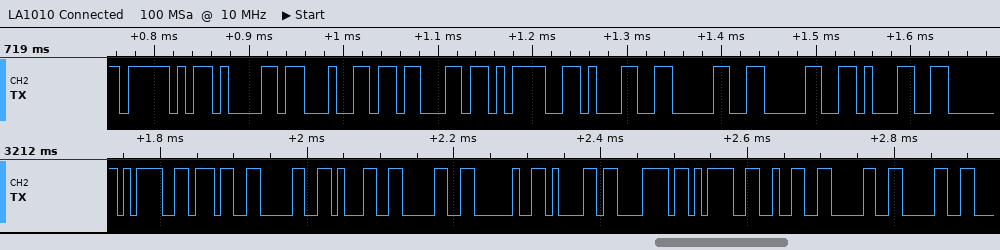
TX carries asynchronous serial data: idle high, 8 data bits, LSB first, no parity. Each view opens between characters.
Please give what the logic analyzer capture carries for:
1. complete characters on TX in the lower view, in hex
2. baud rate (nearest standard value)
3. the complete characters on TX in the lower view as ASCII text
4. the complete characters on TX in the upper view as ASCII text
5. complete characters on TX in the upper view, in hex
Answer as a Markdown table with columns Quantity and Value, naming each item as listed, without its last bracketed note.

| Quantity | Value |
|---|---|
| complete characters on TX in the lower view, in hex | 3D, 37, 30, 31, 30, 20, 61, 78, 3D, 32, 30, 30 |
| baud rate | 115200 baud |
| the complete characters on TX in the lower view as ASCII text | "=7010 ax=200" |
| the complete characters on TX in the upper view as ASCII text | "_adc=1001" |
| complete characters on TX in the upper view, in hex | 5F, 61, 64, 63, 3D, 31, 30, 30, 31 |
